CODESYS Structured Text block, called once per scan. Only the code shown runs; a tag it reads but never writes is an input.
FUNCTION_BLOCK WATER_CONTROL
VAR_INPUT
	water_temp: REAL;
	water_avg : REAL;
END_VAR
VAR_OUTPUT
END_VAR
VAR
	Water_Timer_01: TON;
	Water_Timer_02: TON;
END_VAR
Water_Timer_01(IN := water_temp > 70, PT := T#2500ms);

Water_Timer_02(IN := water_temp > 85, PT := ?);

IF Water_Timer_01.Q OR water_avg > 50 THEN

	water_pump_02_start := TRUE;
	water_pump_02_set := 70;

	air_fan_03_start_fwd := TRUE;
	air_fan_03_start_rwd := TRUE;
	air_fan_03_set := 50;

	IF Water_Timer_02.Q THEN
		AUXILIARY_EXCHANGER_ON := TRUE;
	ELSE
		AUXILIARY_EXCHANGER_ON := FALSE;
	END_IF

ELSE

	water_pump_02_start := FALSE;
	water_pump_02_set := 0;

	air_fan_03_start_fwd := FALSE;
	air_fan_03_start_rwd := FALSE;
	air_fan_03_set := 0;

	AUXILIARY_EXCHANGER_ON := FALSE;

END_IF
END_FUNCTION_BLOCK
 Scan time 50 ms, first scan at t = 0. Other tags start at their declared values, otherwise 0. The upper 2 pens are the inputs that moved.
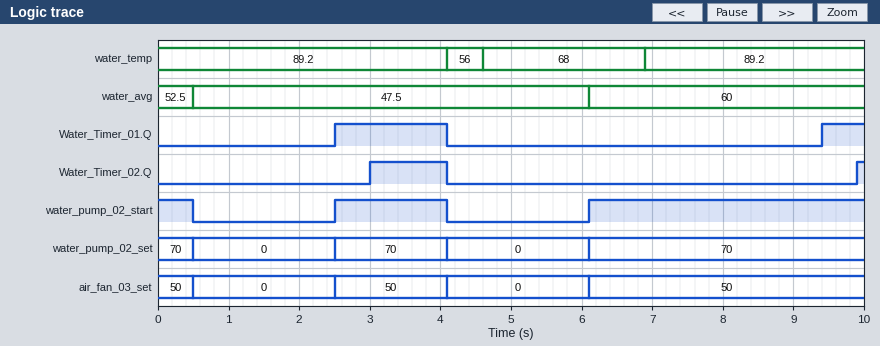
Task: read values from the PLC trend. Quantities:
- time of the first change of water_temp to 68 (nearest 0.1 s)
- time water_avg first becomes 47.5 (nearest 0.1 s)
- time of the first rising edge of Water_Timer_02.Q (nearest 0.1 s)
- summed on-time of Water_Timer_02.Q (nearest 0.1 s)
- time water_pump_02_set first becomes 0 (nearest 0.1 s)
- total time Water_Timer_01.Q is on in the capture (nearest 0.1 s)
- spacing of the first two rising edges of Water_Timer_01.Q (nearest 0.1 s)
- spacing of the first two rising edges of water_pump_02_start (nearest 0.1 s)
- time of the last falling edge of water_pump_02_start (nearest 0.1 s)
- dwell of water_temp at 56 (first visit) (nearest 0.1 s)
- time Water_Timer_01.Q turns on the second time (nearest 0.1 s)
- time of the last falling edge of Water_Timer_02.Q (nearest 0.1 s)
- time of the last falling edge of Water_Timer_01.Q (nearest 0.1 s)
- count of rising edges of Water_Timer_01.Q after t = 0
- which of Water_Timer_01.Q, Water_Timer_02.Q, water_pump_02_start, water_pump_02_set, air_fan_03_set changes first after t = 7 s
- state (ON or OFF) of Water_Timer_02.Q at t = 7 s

4.6 s
0.5 s
3.0 s
1.2 s
0.5 s
2.2 s
6.9 s
3.6 s
4.1 s
0.5 s
9.4 s
4.1 s
4.1 s
2
Water_Timer_01.Q
OFF
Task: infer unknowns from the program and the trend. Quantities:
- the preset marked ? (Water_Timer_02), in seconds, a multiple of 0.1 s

3.0 s
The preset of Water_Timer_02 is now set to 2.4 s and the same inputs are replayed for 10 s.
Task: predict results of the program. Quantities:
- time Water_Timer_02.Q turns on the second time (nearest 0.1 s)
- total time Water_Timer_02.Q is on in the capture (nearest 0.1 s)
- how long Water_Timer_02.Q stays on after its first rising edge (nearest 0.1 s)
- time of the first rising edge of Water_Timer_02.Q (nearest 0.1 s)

9.3 s
2.4 s
1.7 s
2.4 s
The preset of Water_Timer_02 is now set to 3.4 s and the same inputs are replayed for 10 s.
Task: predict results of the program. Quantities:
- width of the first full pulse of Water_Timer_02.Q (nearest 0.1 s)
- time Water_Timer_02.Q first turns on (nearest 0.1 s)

0.7 s
3.4 s
